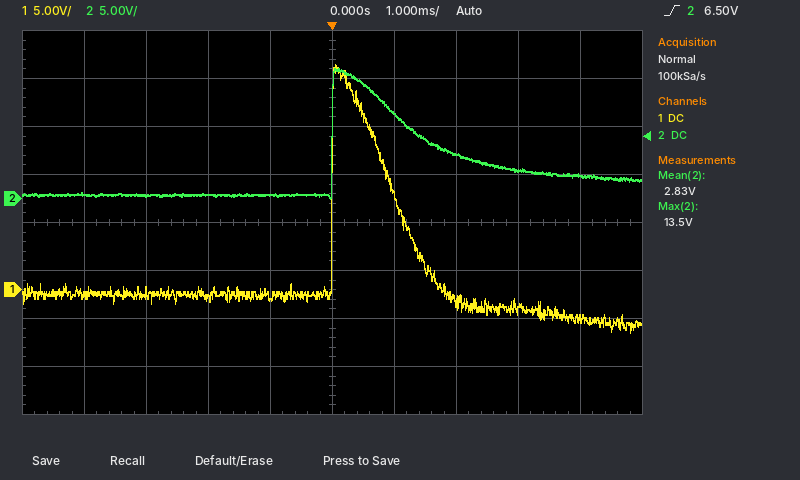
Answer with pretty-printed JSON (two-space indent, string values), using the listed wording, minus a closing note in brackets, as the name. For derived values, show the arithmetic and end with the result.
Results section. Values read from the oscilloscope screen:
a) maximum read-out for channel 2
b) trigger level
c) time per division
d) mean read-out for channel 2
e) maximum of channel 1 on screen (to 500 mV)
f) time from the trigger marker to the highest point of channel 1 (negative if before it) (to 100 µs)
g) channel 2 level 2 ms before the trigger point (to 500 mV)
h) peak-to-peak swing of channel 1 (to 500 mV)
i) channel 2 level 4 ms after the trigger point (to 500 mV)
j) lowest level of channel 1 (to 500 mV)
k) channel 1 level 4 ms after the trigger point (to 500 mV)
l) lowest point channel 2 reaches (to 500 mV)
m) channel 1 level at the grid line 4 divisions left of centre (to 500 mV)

{
  "maximum read-out for channel 2": "13.5 V",
  "trigger level": "6.50 V",
  "time per division": "1 ms",
  "mean read-out for channel 2": "2.83 V",
  "maximum of channel 1 on screen": "23.5 V",
  "time from the trigger marker to the highest point of channel 1 (negative if before it)": "+100 µs",
  "channel 2 level 2 ms before the trigger point": "500 mV",
  "peak-to-peak swing of channel 1": "23.5 V − (-4.5 V) = 28.0 V",
  "channel 2 level 4 ms after the trigger point": "2.5 V",
  "lowest level of channel 1": "-4.5 V",
  "channel 1 level 4 ms after the trigger point": "-3.0 V",
  "lowest point channel 2 reaches": "0.0 V",
  "channel 1 level at the grid line 4 divisions left of centre": "-500 mV"
}
